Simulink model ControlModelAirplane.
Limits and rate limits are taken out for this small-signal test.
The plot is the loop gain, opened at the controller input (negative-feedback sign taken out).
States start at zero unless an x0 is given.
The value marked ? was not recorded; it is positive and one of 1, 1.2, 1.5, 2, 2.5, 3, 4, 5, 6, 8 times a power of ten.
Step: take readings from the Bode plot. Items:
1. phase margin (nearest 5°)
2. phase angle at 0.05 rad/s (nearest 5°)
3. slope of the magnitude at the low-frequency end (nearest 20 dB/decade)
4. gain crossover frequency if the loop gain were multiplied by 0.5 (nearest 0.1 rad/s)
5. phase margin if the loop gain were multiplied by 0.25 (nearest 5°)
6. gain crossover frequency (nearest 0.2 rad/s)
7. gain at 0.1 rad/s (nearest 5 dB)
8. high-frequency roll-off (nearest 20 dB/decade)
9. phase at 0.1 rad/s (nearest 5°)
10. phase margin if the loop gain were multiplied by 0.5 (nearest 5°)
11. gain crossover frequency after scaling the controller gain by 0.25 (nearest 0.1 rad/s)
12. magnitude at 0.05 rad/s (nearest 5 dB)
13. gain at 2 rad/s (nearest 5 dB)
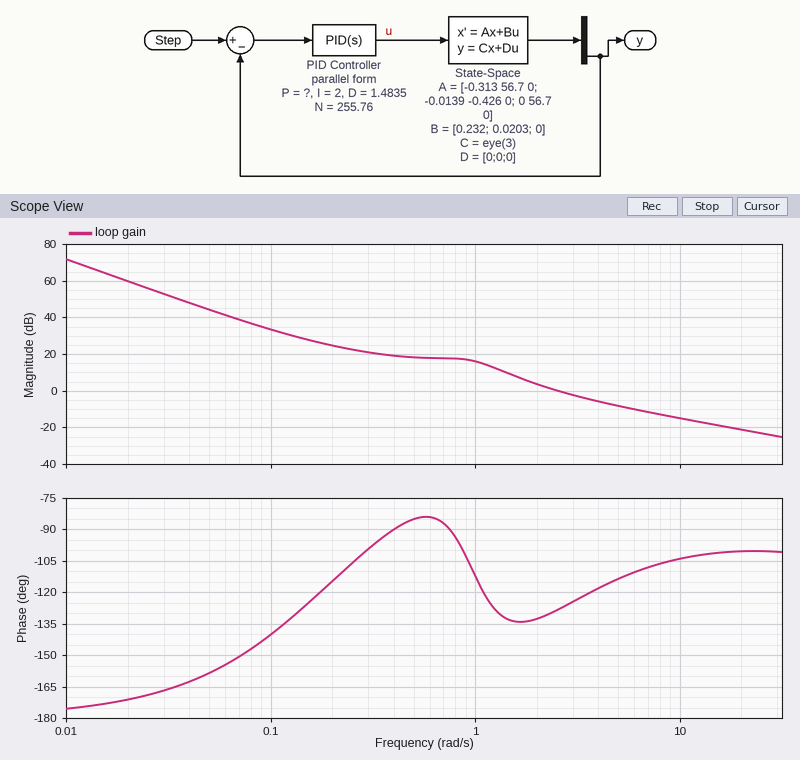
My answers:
50°
-160°
-40 dB/decade
1.7 rad/s
50°
2.6 rad/s
35 dB
-20 dB/decade
-140°
45°
1.3 rad/s
45 dB
5 dB
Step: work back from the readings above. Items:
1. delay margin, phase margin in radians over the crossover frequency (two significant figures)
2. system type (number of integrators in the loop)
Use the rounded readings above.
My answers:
0.34 s
2
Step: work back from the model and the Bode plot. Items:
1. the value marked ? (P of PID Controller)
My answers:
4
